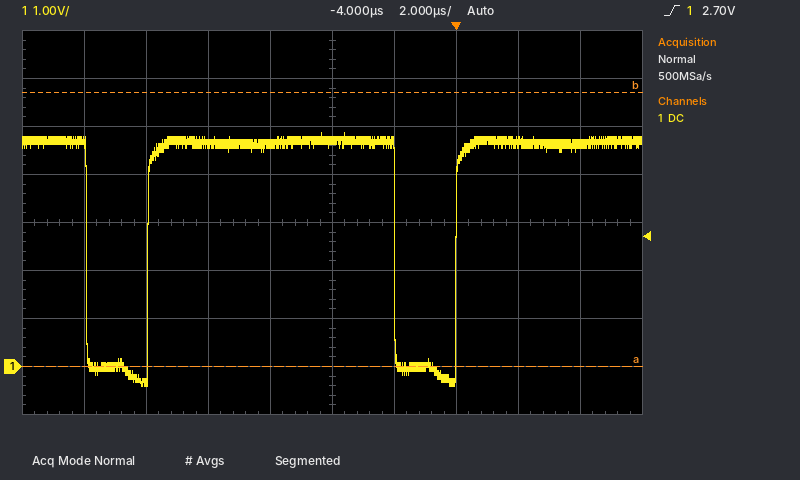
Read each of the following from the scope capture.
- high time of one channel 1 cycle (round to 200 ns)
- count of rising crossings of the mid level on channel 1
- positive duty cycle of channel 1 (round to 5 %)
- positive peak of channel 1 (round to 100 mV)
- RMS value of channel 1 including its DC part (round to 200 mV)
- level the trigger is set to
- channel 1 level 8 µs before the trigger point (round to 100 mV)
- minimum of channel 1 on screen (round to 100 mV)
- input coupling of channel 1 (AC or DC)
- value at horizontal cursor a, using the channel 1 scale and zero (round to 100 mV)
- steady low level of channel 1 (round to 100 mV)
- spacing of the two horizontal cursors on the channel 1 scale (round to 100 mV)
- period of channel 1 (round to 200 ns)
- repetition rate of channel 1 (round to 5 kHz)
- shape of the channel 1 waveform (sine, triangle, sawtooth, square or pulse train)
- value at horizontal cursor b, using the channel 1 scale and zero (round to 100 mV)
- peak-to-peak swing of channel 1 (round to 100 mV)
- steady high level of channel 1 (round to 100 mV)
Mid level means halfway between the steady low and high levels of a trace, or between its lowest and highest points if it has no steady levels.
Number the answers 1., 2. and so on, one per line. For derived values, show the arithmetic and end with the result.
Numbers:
1. 8.0 µs
2. 2
3. 8.0 µs / 10.0 µs ≈ 80 %
4. 4.9 V
5. √(0.8 × (4.7 V)² + 0.2 × (0.0 V)²) ≈ 4.2 V
6. 2.70 V
7. 4.6 V
8. -400 mV
9. DC
10. 0.0 V
11. 0.0 V
12. 5.7 V
13. 10.0 µs
14. 1 / 10.0 µs ≈ 100 kHz
15. pulse train
16. 5.7 V
17. 4.9 V − (-400 mV) = 5.3 V
18. 4.7 V
